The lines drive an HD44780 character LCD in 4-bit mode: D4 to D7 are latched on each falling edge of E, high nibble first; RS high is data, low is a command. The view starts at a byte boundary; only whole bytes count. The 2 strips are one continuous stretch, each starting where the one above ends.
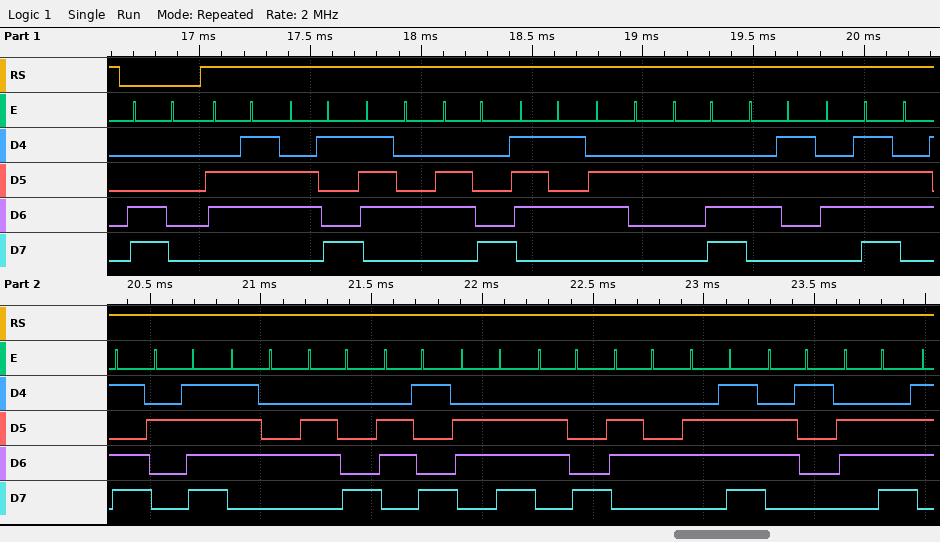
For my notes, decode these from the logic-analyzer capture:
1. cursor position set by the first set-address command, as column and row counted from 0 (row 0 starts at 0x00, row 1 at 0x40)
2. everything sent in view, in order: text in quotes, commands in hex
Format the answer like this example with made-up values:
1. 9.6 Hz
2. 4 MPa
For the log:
1. column 0, row 1
2. 0xC0 "github.com/thinhdoan"
